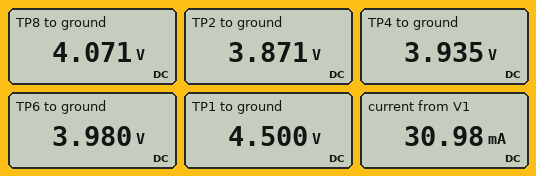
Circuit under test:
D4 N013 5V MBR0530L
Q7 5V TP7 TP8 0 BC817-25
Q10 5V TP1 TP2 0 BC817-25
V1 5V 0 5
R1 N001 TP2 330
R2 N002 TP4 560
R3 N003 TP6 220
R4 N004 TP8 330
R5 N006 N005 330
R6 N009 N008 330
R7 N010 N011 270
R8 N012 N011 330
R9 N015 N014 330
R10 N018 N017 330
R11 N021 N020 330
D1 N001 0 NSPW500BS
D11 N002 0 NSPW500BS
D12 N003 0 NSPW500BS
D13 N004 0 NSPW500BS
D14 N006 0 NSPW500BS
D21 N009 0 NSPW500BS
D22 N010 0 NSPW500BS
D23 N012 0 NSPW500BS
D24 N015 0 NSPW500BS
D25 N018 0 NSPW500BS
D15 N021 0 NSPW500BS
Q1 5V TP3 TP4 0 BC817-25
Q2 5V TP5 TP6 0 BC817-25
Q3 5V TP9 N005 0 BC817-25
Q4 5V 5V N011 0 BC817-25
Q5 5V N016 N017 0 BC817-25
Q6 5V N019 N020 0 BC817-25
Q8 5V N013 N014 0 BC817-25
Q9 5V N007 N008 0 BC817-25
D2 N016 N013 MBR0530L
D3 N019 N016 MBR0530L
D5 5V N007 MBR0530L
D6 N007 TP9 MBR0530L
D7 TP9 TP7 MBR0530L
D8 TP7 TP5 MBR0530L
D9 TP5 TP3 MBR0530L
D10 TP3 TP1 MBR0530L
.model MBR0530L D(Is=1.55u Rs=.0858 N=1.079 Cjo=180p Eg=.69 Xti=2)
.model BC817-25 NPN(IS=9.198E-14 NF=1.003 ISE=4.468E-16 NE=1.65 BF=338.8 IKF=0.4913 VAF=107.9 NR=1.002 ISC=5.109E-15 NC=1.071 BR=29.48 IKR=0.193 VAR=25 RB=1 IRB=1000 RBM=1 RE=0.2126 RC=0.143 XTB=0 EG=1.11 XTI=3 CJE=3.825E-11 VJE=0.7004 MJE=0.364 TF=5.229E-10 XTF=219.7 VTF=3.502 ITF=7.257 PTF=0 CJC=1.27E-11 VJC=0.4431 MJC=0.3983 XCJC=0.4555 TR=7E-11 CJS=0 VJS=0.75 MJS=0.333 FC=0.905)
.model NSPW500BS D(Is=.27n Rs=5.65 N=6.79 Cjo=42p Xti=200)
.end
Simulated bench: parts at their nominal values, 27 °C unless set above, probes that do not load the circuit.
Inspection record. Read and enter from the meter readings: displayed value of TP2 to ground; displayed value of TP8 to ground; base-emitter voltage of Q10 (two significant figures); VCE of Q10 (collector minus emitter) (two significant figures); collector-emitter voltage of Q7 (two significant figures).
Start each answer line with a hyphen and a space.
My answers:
- 3.871 V
- 4.071 V
- 630 mV
- 1.1 V
- 930 mV
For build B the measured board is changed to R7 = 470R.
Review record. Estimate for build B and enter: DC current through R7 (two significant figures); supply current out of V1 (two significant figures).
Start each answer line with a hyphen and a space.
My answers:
- 3.1 mA
- 29 mA
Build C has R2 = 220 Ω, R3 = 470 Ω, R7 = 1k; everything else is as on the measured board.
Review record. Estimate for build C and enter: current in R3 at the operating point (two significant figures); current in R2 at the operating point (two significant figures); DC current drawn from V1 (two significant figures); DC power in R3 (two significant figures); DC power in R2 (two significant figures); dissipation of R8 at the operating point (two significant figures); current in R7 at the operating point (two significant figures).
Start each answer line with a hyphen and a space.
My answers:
- 2.5 mA
- 4.4 mA
- 28 mA
- 2.9 mW
- 4.2 mW
- 6.1 mW
- 1.6 mA
